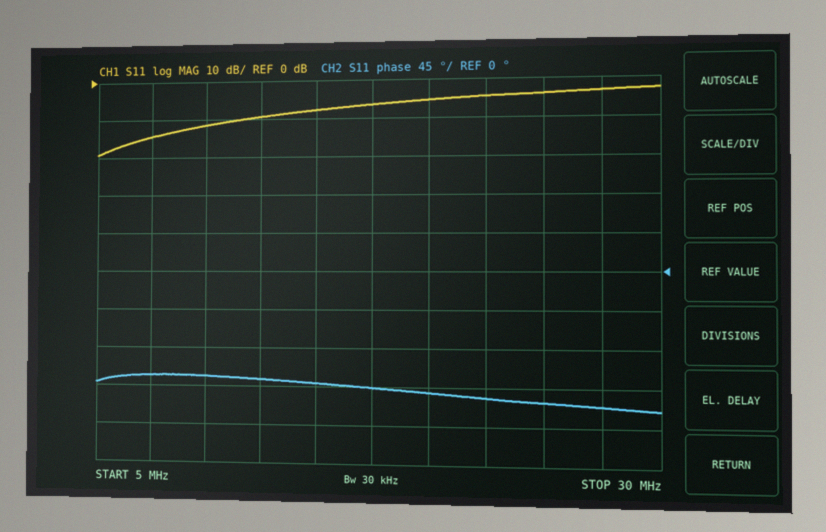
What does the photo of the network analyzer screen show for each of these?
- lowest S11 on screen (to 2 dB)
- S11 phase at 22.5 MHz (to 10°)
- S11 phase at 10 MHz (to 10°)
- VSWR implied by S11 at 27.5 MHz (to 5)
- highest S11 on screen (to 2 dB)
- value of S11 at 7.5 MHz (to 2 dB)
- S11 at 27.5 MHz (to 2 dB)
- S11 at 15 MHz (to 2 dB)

-20 dB
-150°
-120°
5
-2 dB
-14 dB
-4 dB
-8 dB
